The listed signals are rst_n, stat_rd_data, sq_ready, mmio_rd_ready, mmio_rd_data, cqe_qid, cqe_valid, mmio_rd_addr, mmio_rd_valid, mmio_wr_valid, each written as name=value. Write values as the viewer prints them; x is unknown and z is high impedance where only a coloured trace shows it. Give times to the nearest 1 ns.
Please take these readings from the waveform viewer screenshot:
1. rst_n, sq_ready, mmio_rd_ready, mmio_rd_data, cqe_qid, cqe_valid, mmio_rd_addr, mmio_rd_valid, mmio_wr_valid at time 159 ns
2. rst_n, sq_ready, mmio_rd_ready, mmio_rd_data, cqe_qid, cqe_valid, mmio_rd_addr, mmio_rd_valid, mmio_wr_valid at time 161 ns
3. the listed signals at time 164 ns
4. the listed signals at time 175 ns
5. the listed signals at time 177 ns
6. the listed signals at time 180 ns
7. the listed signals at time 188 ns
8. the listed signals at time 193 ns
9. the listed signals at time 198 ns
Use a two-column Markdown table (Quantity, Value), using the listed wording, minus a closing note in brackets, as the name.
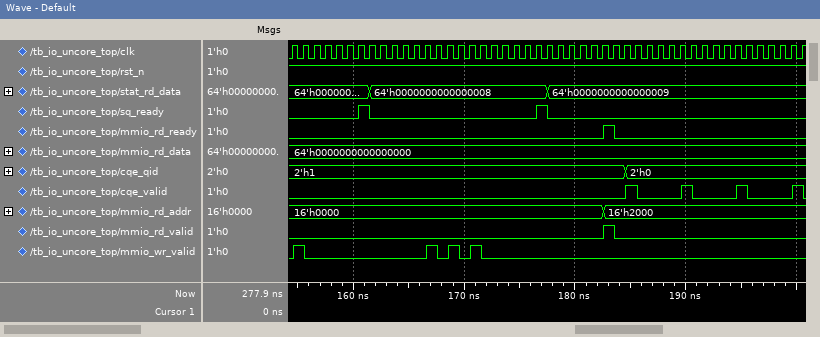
| Quantity | Value |
|---|---|
| rst_n, sq_ready, mmio_rd_ready, mmio_rd_data, cqe_qid, cqe_valid, mmio_rd_addr, mmio_rd_valid, mmio_wr_valid at time 159 ns | rst_n=1, sq_ready=0, mmio_rd_ready=0, mmio_rd_data=64'h0000000000000000, cqe_qid=2'h1, cqe_valid=0, mmio_rd_addr=16'h0000, mmio_rd_valid=0, mmio_wr_valid=0 |
| rst_n, sq_ready, mmio_rd_ready, mmio_rd_data, cqe_qid, cqe_valid, mmio_rd_addr, mmio_rd_valid, mmio_wr_valid at time 161 ns | rst_n=1, sq_ready=1, mmio_rd_ready=0, mmio_rd_data=64'h0000000000000000, cqe_qid=2'h1, cqe_valid=0, mmio_rd_addr=16'h0000, mmio_rd_valid=0, mmio_wr_valid=0 |
| the listed signals at time 164 ns | rst_n=1, stat_rd_data=64'h0000000000000008, sq_ready=0, mmio_rd_ready=0, mmio_rd_data=64'h0000000000000000, cqe_qid=2'h1, cqe_valid=0, mmio_rd_addr=16'h0000, mmio_rd_valid=0, mmio_wr_valid=0 |
| the listed signals at time 175 ns | rst_n=1, stat_rd_data=64'h0000000000000008, sq_ready=0, mmio_rd_ready=0, mmio_rd_data=64'h0000000000000000, cqe_qid=2'h1, cqe_valid=0, mmio_rd_addr=16'h0000, mmio_rd_valid=0, mmio_wr_valid=0 |
| the listed signals at time 177 ns | rst_n=1, stat_rd_data=64'h0000000000000008, sq_ready=1, mmio_rd_ready=0, mmio_rd_data=64'h0000000000000000, cqe_qid=2'h1, cqe_valid=0, mmio_rd_addr=16'h0000, mmio_rd_valid=0, mmio_wr_valid=0 |
| the listed signals at time 180 ns | rst_n=1, stat_rd_data=64'h0000000000000009, sq_ready=0, mmio_rd_ready=0, mmio_rd_data=64'h0000000000000000, cqe_qid=2'h1, cqe_valid=0, mmio_rd_addr=16'h0000, mmio_rd_valid=0, mmio_wr_valid=0 |
| the listed signals at time 188 ns | rst_n=1, stat_rd_data=64'h0000000000000009, sq_ready=0, mmio_rd_ready=0, mmio_rd_data=64'h0000000000000000, cqe_qid=2'h0, cqe_valid=0, mmio_rd_addr=16'h2000, mmio_rd_valid=0, mmio_wr_valid=0 |
| the listed signals at time 193 ns | rst_n=1, stat_rd_data=64'h0000000000000009, sq_ready=0, mmio_rd_ready=0, mmio_rd_data=64'h0000000000000000, cqe_qid=2'h0, cqe_valid=0, mmio_rd_addr=16'h2000, mmio_rd_valid=0, mmio_wr_valid=0 |
| the listed signals at time 198 ns | rst_n=1, stat_rd_data=64'h0000000000000009, sq_ready=0, mmio_rd_ready=0, mmio_rd_data=64'h0000000000000000, cqe_qid=2'h0, cqe_valid=0, mmio_rd_addr=16'h2000, mmio_rd_valid=0, mmio_wr_valid=0 |
